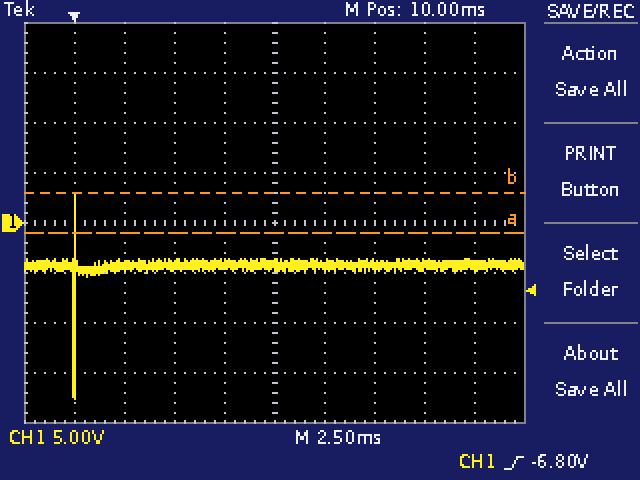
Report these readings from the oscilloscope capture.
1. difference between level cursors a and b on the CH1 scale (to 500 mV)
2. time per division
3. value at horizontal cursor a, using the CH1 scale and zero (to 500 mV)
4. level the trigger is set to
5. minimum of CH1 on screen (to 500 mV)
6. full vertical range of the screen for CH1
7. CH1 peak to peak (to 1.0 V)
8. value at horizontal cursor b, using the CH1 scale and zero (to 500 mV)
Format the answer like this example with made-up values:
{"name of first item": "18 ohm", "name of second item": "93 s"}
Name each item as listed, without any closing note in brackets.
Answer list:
{"difference between level cursors a and b on the CH1 scale": "4.0 V", "time per division": "2.5 ms", "value at horizontal cursor a, using the CH1 scale and zero": "-1.0 V", "level the trigger is set to": "-6.80 V", "minimum of CH1 on screen": "-17.5 V", "full vertical range of the screen for CH1": "40 V", "CH1 peak to peak": "20.0 V", "value at horizontal cursor b, using the CH1 scale and zero": "3.0 V"}
